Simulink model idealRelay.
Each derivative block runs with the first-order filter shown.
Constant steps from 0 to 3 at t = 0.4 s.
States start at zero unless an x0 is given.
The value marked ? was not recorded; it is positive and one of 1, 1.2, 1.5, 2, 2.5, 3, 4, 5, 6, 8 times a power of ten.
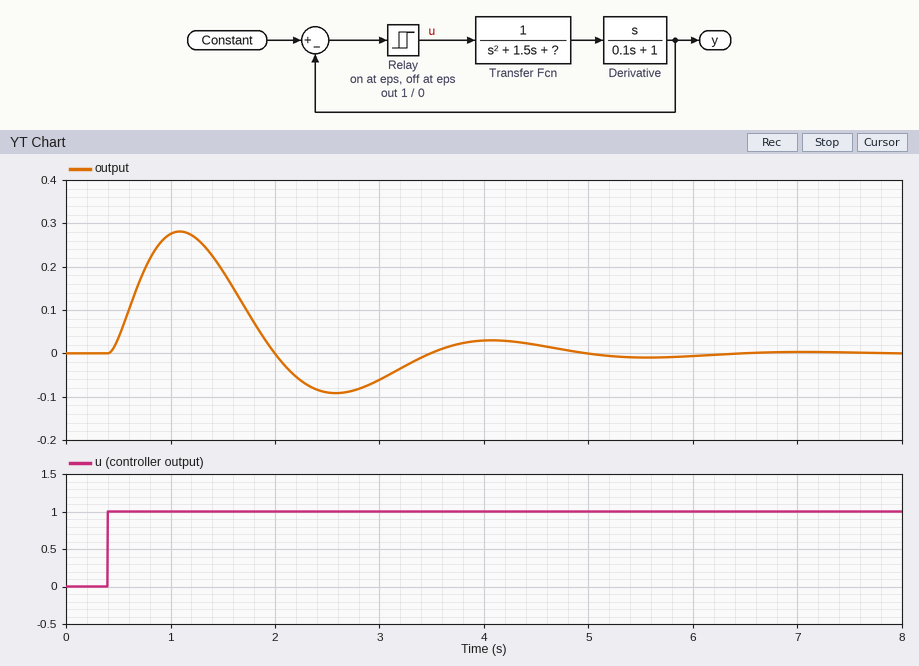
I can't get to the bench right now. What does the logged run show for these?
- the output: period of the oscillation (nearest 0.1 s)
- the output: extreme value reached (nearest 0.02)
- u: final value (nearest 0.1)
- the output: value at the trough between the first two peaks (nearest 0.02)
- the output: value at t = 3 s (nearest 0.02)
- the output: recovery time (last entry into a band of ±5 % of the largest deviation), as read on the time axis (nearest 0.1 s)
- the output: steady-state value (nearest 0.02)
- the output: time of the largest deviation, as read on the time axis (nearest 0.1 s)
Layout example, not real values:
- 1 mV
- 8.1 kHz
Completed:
- 3.0 s
- 0.28
- 1.0
- -0.10
- -0.06
- 4.6 s
- 0.00
- 1.1 s
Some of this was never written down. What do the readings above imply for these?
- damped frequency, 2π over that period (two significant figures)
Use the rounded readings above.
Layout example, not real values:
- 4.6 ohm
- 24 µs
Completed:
- 2.1 rad/s
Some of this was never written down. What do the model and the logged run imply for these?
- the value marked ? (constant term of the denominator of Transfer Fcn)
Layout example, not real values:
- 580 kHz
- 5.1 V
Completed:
- 5
